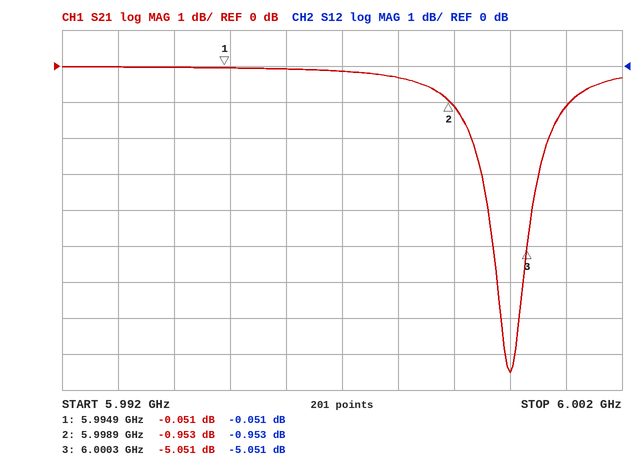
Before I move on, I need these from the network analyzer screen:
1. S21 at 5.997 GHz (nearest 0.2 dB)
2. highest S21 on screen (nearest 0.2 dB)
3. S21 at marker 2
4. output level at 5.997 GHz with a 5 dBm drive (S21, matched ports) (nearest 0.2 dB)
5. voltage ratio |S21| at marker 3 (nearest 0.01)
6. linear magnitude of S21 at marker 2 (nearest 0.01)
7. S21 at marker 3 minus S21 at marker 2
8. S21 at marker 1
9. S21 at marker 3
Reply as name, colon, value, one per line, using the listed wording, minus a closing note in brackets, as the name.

S21 at 5.997 GHz: -0.2 dB
highest S21 on screen: 0.0 dB
S21 at marker 2: -0.953 dB
output level at 5.997 GHz with a 5 dBm drive (S21, matched ports): 4.8 dBm
voltage ratio |S21| at marker 3: 0.56
linear magnitude of S21 at marker 2: 0.90
S21 at marker 3 minus S21 at marker 2: -4.098 dB
S21 at marker 1: -0.051 dB
S21 at marker 3: -5.051 dB
